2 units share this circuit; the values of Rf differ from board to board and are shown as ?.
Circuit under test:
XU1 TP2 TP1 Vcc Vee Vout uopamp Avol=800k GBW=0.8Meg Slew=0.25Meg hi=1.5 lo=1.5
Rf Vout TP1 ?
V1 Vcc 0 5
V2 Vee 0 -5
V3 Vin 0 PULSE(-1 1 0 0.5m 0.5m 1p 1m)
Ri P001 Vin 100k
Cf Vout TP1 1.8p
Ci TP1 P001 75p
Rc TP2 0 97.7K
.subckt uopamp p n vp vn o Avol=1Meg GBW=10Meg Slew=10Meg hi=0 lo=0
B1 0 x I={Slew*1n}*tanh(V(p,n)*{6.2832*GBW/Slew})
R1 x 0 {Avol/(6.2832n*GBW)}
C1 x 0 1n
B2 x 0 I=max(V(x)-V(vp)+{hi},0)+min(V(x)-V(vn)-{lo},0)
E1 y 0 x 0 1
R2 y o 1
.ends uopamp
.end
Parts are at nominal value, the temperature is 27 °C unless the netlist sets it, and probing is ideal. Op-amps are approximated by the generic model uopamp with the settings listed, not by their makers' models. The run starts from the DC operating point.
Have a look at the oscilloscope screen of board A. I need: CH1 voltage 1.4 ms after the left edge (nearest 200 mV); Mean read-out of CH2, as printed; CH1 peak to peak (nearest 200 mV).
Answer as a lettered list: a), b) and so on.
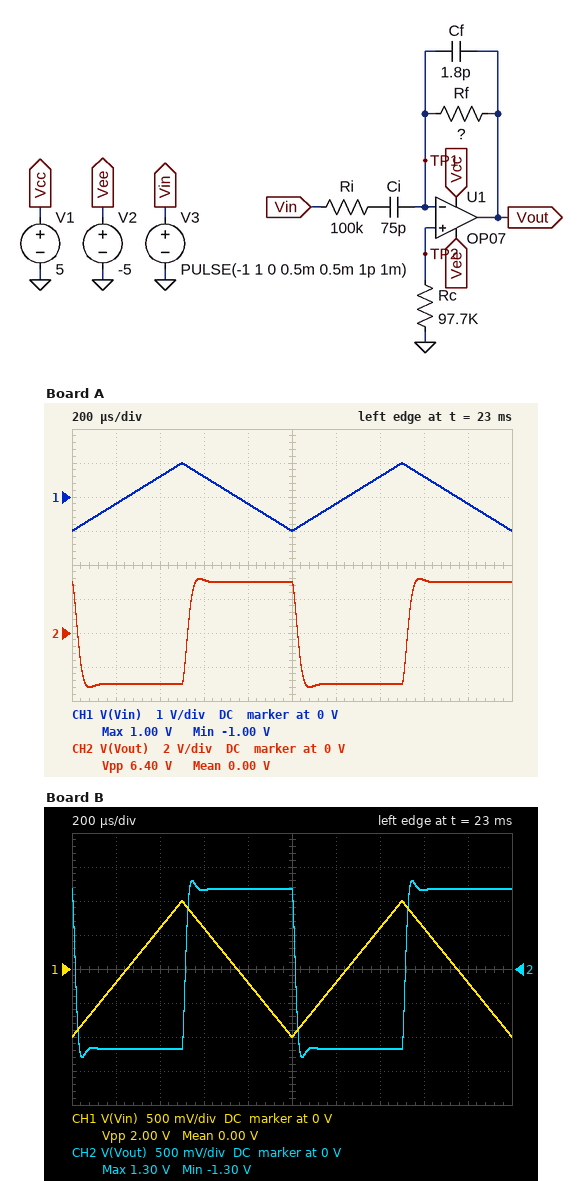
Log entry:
a) 600 mV
b) 0.00 V
c) 2.0 V
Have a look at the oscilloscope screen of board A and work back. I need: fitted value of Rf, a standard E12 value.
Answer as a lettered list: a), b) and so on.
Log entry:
a) 10 MΩ
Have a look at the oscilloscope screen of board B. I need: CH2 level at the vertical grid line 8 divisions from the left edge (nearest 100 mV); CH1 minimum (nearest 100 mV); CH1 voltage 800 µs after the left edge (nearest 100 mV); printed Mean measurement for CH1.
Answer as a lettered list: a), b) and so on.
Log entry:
a) 1.2 V
b) -1.0 V
c) -200 mV
d) 0.00 V
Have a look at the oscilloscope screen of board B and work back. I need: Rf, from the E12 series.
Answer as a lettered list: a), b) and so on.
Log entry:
a) 3.9 MΩ
